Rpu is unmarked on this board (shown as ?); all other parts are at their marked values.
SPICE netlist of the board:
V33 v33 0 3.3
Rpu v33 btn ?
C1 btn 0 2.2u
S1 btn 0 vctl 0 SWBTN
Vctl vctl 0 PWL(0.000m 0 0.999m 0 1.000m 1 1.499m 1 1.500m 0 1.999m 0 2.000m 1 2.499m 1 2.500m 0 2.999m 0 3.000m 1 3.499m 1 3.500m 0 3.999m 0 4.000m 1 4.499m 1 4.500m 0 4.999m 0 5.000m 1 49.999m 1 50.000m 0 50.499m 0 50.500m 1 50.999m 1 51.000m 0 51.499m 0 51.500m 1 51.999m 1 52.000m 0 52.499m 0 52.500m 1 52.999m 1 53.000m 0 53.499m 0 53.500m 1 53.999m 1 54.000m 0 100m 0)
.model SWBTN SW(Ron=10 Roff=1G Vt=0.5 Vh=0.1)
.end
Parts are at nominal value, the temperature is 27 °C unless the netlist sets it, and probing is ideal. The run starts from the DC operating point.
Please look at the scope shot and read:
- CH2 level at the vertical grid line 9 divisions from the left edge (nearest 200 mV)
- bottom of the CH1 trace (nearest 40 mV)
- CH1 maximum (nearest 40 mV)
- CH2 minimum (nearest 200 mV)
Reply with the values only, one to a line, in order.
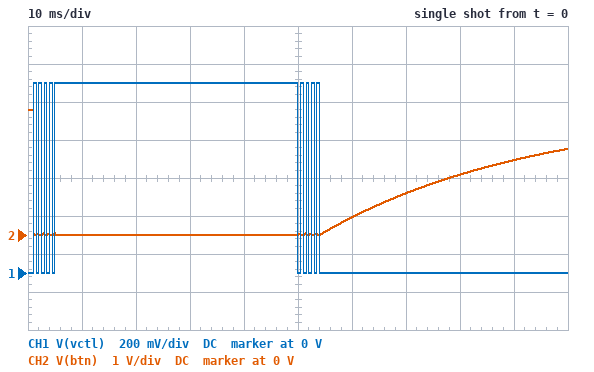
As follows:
2.0 V
0 V
1.00 V
0 V
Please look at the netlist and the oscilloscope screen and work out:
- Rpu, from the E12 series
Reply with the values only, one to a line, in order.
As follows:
18 kΩ
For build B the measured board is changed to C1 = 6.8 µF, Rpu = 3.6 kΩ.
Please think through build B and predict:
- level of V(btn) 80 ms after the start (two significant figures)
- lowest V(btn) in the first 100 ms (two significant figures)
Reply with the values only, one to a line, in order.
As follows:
2.2 V
9.1 mV
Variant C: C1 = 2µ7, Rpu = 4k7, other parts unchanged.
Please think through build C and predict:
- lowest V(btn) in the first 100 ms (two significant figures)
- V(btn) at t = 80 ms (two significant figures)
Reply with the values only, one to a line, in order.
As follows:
7.0 mV
2.9 V
